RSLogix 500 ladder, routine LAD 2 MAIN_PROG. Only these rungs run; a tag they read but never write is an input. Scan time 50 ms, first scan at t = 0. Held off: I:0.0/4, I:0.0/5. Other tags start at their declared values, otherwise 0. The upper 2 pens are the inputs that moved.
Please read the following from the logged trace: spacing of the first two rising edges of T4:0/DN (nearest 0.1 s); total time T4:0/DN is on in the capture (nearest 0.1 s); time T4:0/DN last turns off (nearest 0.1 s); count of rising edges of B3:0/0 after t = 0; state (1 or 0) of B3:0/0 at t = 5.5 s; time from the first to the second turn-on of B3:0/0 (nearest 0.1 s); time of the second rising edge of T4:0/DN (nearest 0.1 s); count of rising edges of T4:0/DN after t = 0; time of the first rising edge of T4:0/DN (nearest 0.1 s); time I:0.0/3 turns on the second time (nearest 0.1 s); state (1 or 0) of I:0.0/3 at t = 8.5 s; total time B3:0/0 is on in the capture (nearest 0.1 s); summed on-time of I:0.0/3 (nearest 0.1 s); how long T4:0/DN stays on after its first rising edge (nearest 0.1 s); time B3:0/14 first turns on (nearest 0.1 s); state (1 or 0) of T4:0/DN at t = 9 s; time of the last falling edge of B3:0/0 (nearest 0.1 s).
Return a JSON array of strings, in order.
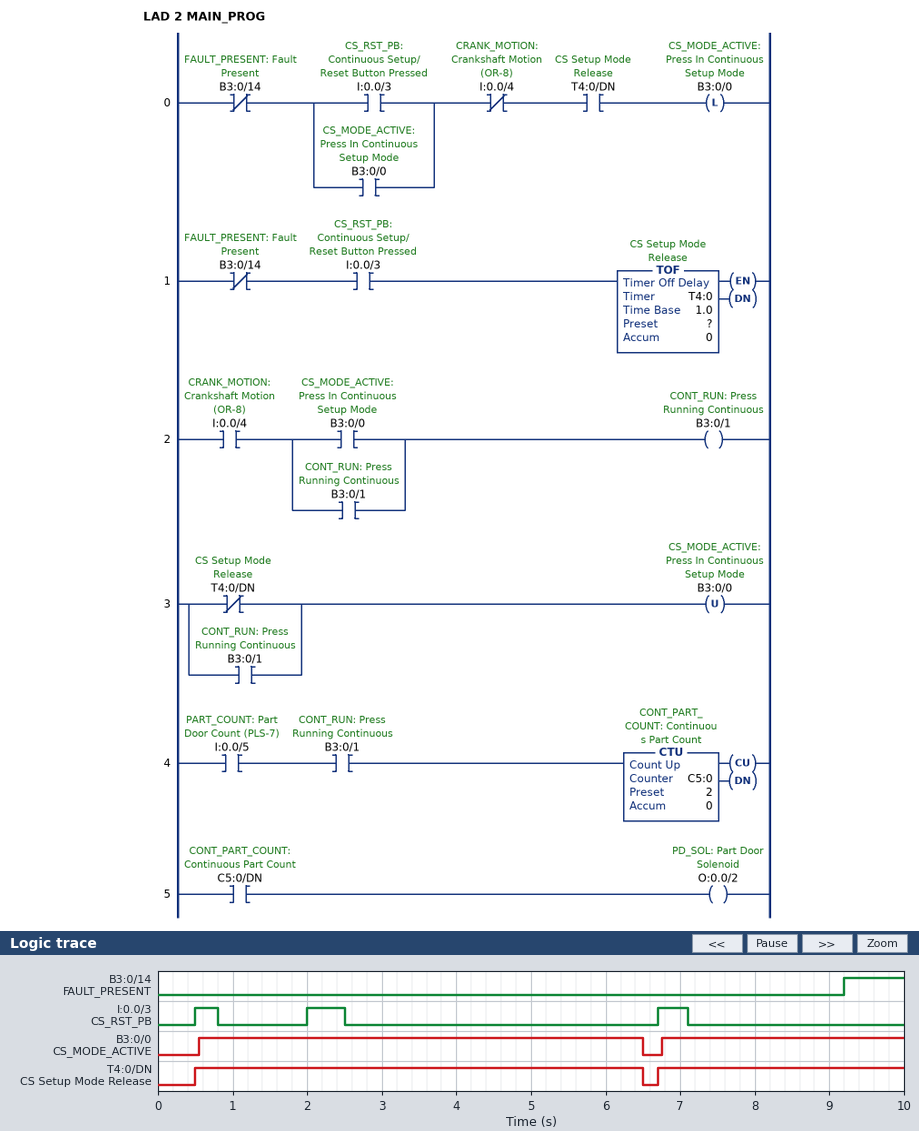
["6.2 s", "9.3 s", "6.5 s", "2", "1", "6.2 s", "6.7 s", "2", "0.5 s", "2.0 s", "0", "9.2 s", "1.2 s", "6.0 s", "9.2 s", "1", "6.5 s"]
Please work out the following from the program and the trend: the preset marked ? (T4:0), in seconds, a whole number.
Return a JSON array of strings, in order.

["4 s"]
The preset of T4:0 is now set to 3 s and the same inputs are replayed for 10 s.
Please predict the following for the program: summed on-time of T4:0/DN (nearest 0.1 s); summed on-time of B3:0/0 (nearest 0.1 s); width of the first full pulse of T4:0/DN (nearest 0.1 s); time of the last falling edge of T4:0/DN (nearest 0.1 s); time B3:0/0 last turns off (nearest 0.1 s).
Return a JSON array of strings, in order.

["8.3 s", "8.2 s", "5.0 s", "5.5 s", "5.5 s"]
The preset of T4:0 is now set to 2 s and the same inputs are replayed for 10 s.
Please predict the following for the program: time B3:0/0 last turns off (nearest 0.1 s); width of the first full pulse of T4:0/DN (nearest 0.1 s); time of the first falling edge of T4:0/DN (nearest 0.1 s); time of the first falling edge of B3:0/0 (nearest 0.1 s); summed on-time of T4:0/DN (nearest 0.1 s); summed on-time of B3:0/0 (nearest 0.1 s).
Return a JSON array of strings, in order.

["9.1 s", "4.0 s", "4.5 s", "4.5 s", "6.4 s", "6.3 s"]
